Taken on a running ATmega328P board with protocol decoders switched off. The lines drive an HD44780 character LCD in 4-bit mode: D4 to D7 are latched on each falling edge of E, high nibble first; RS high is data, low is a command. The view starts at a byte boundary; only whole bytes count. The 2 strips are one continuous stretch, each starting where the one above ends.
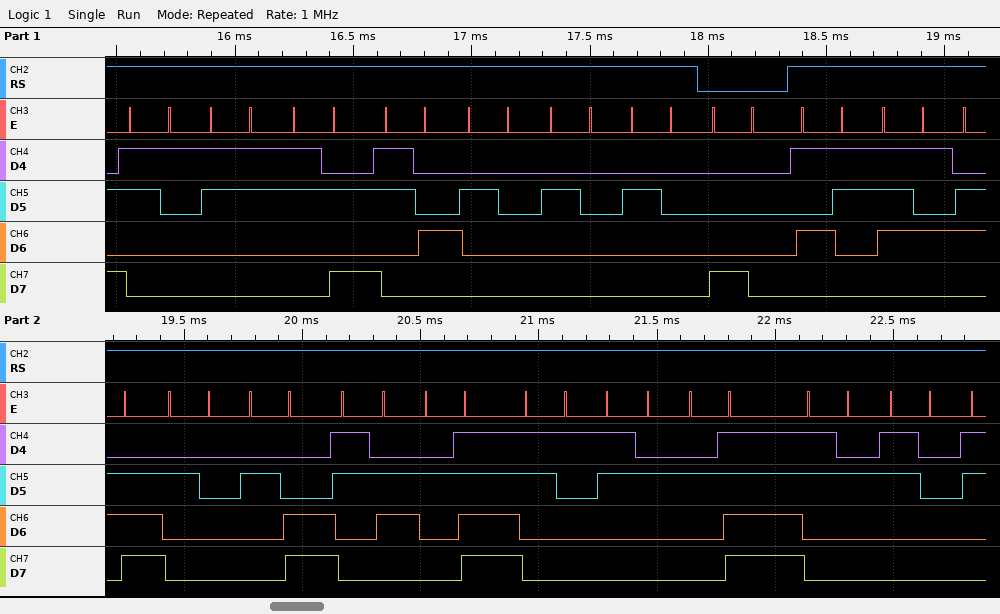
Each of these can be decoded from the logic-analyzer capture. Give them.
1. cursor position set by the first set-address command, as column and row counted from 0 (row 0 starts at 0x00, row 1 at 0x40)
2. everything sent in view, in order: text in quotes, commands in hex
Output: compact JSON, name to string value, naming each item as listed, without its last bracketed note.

{"cursor position set by the first set-address command, as column and row counted from 0": "column 0, row 0", "everything sent in view, in order: text in quotes, commands in hex": "\"13:4   \" 0x80 \"Sun ,6/12/20\""}
